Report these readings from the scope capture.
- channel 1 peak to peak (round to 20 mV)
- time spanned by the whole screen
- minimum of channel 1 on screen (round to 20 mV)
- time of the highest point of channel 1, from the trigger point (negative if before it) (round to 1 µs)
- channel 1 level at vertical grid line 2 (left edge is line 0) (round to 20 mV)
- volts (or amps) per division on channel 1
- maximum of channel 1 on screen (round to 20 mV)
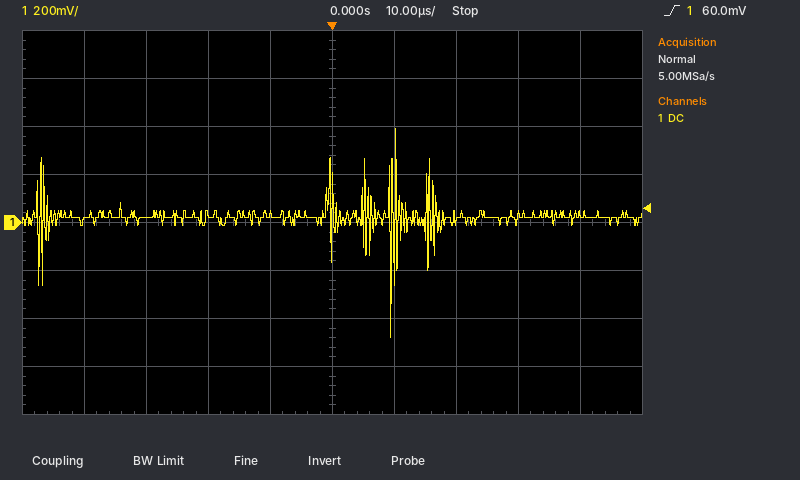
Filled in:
880 mV
100 µs
-480 mV
+10 µs
20 mV
200 mV
400 mV
